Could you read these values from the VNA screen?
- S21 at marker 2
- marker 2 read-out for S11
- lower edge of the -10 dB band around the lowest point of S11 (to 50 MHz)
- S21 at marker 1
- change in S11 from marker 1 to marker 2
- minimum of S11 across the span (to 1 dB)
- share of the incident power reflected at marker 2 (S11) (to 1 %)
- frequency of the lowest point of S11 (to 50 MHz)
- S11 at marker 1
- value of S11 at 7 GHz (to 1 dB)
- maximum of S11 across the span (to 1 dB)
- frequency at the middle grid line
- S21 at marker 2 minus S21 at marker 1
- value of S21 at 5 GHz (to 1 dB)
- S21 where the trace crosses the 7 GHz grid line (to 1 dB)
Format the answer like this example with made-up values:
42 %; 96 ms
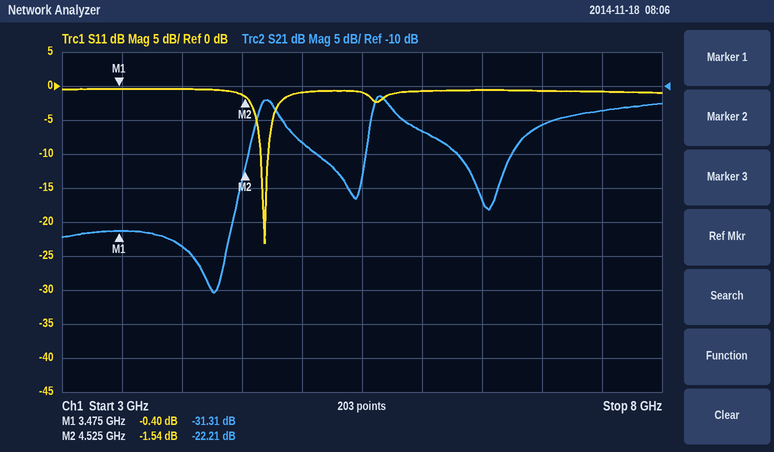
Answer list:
-22.21 dB; -1.54 dB; 4.65 GHz; -31.31 dB; -1.14 dB; -23 dB; 70 %; 4.70 GHz; -0.40 dB; -1 dB; 0 dB; 5.5 GHz; 9.10 dB; -18 dB; -16 dB
